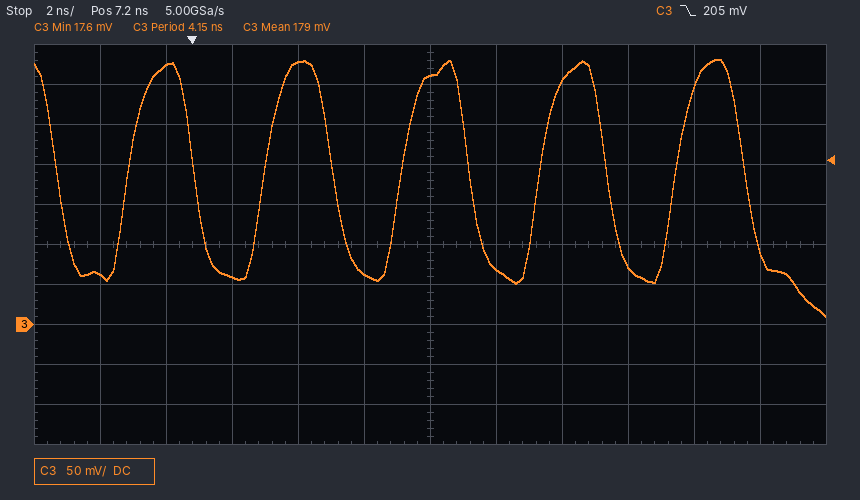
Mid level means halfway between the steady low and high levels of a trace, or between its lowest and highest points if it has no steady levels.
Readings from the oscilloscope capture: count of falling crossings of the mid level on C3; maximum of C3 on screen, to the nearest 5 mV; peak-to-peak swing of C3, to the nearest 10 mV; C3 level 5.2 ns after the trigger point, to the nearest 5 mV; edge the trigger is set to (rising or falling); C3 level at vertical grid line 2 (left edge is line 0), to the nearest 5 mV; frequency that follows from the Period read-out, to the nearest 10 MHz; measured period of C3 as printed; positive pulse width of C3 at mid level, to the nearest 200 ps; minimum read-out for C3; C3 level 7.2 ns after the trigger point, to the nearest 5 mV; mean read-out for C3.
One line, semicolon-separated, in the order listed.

6; 330 mV; 320 mV; 65 mV; falling; 325 mV; 240 MHz; 4.15 ns; 2.2 ns; 17.6 mV; 310 mV; 179 mV
